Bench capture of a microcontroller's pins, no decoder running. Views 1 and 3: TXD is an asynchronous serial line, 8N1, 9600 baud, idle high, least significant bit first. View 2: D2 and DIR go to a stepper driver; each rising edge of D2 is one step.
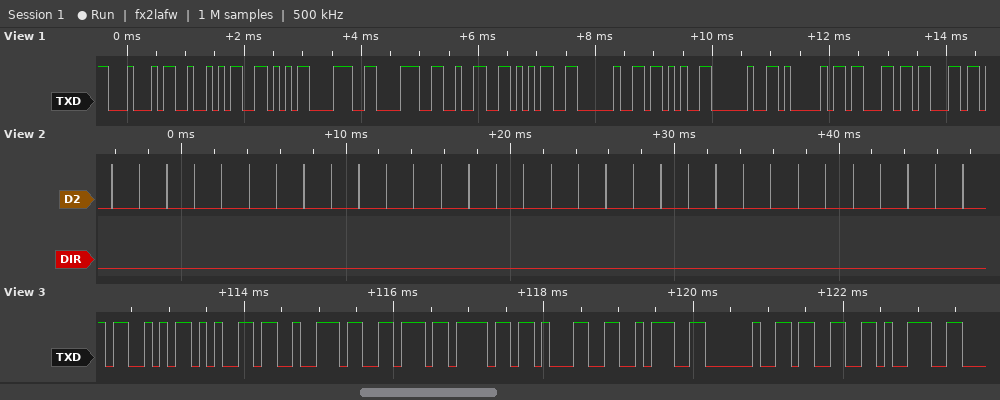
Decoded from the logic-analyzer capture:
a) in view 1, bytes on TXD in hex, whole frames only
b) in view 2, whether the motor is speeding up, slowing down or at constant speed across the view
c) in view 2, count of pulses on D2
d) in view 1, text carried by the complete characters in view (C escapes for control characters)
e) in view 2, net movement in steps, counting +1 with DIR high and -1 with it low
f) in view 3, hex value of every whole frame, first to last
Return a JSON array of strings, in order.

["44 52 56 38 38 32 35 20 2B 20 41 63 63", "constant speed", "32", "\"DRV8825 + Acc\"", "-32", "0x53 0x65 0x72 0x76 0x6F 0x31 0x3A 0x20 0x33 0x39"]
